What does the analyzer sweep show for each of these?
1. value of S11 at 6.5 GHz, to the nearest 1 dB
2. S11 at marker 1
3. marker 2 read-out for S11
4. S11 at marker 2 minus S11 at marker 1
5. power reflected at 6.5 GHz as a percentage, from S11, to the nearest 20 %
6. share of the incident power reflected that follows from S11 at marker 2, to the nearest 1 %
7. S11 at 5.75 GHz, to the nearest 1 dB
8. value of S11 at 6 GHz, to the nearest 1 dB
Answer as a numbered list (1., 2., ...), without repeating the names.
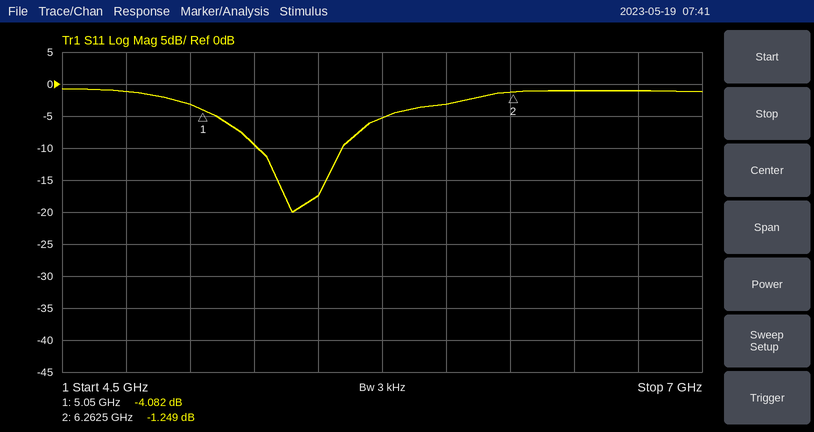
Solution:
1. -1 dB
2. -4.082 dB
3. -1.249 dB
4. 2.833 dB
5. 80 %
6. 75 %
7. -5 dB
8. -3 dB
